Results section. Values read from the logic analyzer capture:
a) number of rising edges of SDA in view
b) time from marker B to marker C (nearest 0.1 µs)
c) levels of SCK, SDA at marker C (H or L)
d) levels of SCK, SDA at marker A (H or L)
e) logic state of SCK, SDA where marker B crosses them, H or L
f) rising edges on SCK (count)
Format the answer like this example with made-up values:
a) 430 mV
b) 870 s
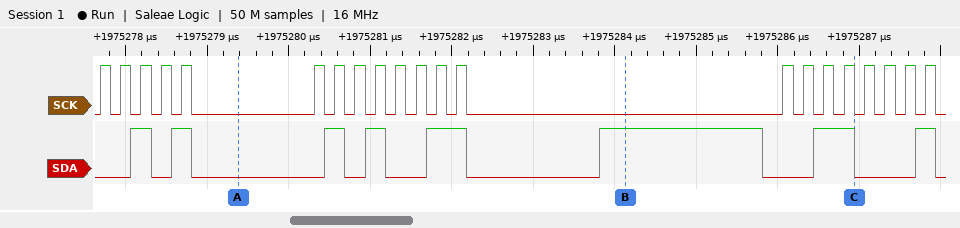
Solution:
a) 8
b) 2.8 µs
c) SCK=L, SDA=L
d) SCK=L, SDA=L
e) SCK=L, SDA=H
f) 21
